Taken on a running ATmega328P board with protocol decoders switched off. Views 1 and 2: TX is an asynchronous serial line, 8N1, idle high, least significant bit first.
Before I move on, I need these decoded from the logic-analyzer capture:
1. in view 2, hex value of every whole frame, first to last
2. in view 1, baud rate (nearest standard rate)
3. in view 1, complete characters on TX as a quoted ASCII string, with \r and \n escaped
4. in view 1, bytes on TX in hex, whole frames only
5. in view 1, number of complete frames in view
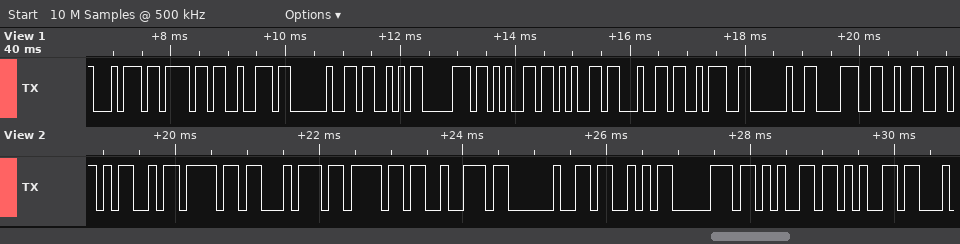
0x4D 0x6F 0x74 0x6F 0x72 0x20 0x53 0x70 0x65 0x65
9600 baud
"tor Speed: 82"
74 6F 72 20 53 70 65 65 64 3A 20 38 32
13
